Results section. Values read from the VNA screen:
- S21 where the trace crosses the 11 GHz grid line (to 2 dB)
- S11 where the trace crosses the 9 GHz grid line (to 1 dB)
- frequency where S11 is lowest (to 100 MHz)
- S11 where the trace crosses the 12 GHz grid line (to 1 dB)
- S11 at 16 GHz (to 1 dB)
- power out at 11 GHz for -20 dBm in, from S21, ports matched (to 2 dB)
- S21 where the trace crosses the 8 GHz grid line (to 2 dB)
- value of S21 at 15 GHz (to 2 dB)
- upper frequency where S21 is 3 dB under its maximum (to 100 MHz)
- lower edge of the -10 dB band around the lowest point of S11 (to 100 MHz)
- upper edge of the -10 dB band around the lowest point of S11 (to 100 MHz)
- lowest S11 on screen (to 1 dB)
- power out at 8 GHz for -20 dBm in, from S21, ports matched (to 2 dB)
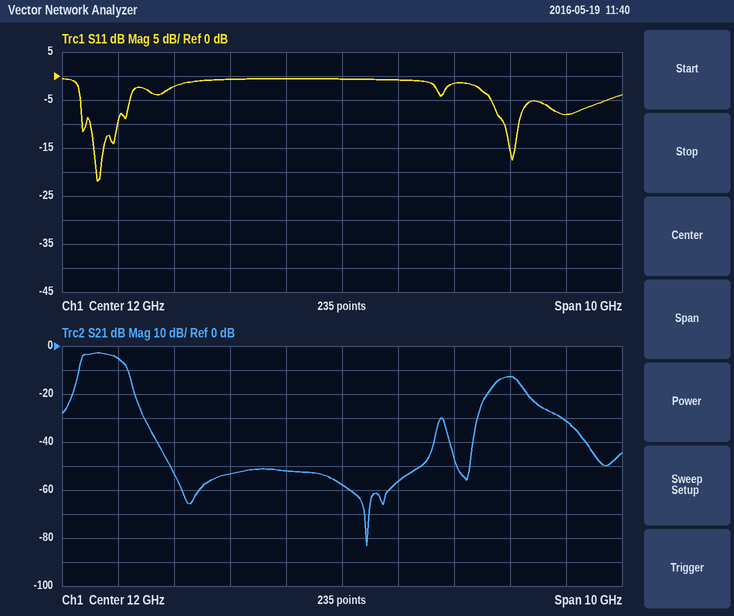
-52 dB
-2 dB
7.6 GHz
-1 dB
-8 dB
-72 dBm
-6 dB
-12 dB
8.0 GHz
7.5 GHz
8.0 GHz
-22 dB
-26 dBm
